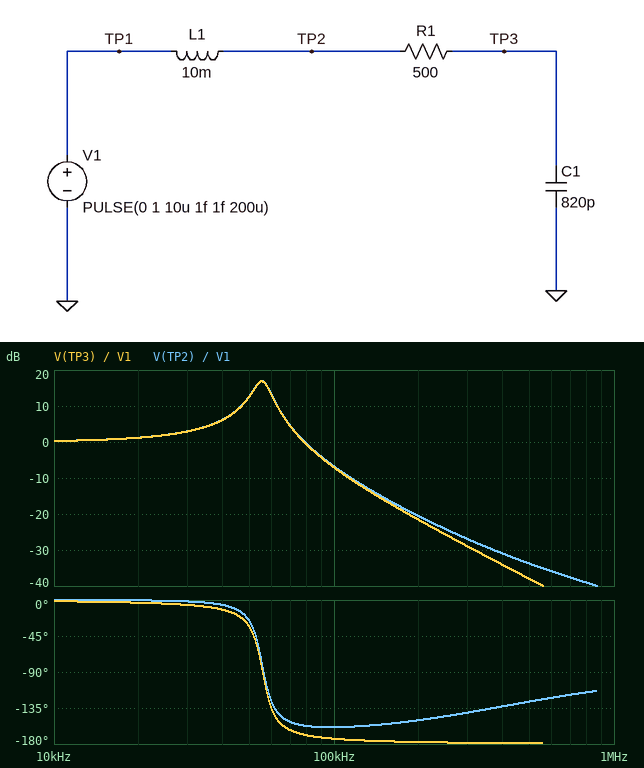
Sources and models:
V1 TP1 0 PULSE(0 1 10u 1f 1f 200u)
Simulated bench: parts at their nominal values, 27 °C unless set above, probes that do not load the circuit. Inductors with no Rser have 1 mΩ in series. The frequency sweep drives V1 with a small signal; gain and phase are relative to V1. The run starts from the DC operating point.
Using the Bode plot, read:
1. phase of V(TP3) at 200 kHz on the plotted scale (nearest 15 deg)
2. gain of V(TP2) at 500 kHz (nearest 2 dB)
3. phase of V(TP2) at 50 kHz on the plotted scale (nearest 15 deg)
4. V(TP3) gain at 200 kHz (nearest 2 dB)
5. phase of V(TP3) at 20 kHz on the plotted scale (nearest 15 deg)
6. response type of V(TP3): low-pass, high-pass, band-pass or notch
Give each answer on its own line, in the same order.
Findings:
-180 deg
-34 dB
-30 deg
-22 dB
0 deg
low-pass
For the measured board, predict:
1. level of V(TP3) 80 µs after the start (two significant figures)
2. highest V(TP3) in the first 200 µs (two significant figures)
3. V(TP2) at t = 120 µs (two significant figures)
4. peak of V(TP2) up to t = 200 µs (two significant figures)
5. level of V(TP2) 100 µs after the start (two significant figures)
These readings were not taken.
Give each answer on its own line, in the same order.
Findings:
880 mV
1.8 V
950 mV
1.8 V
890 mV
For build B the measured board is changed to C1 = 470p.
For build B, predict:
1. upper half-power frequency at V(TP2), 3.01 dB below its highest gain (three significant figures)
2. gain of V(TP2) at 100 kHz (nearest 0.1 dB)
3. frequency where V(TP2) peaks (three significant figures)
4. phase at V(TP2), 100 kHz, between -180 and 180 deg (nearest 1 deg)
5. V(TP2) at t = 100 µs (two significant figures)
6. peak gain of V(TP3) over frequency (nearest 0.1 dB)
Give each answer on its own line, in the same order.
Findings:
77.1 kHz
1.3 dB
73.2 kHz
-162 deg
1.1 V
19.3 dB
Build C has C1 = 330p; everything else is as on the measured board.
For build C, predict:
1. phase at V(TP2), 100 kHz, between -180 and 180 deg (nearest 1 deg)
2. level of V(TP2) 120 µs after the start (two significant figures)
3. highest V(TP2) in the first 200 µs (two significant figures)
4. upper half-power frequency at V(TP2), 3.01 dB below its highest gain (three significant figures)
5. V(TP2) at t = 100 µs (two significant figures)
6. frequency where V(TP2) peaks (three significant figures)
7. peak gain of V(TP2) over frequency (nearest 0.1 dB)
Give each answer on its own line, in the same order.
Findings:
-155 deg
1.0 V
1.9 V
91.3 kHz
920 mV
87.4 kHz
20.9 dB
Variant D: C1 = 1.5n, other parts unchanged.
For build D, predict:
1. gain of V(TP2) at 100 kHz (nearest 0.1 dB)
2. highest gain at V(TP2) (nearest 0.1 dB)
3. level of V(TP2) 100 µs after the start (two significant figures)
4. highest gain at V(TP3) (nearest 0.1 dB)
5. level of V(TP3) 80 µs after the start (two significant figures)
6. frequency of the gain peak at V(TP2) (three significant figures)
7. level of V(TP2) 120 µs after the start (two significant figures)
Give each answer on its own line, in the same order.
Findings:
-13.0 dB
14.5 dB
1.0 V
14.3 dB
900 mV
40.7 kHz
1.1 V
